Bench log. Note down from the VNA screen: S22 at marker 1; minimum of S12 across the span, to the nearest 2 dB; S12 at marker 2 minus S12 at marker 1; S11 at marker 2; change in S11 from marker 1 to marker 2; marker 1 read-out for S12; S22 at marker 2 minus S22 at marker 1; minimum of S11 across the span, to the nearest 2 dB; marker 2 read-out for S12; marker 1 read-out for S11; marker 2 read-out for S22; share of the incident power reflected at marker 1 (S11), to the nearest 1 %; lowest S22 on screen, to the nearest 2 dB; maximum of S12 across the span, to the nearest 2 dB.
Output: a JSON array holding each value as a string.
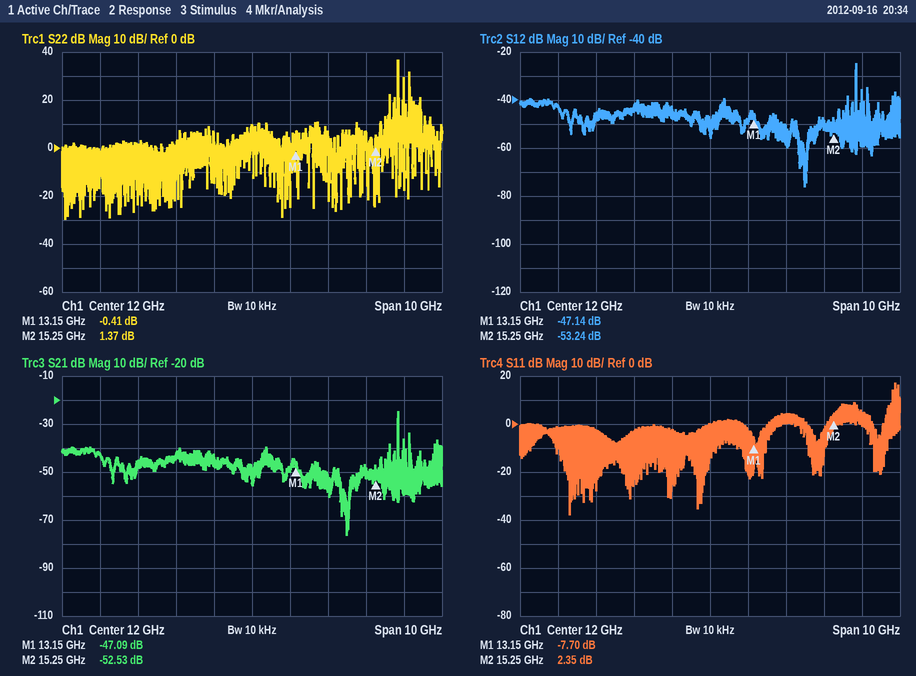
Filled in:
["-0.41 dB", "-76 dB", "-6.10 dB", "2.35 dB", "10.05 dB", "-47.14 dB", "1.78 dB", "-38 dB", "-53.24 dB", "-7.70 dB", "1.37 dB", "17 %", "-30 dB", "-24 dB"]
